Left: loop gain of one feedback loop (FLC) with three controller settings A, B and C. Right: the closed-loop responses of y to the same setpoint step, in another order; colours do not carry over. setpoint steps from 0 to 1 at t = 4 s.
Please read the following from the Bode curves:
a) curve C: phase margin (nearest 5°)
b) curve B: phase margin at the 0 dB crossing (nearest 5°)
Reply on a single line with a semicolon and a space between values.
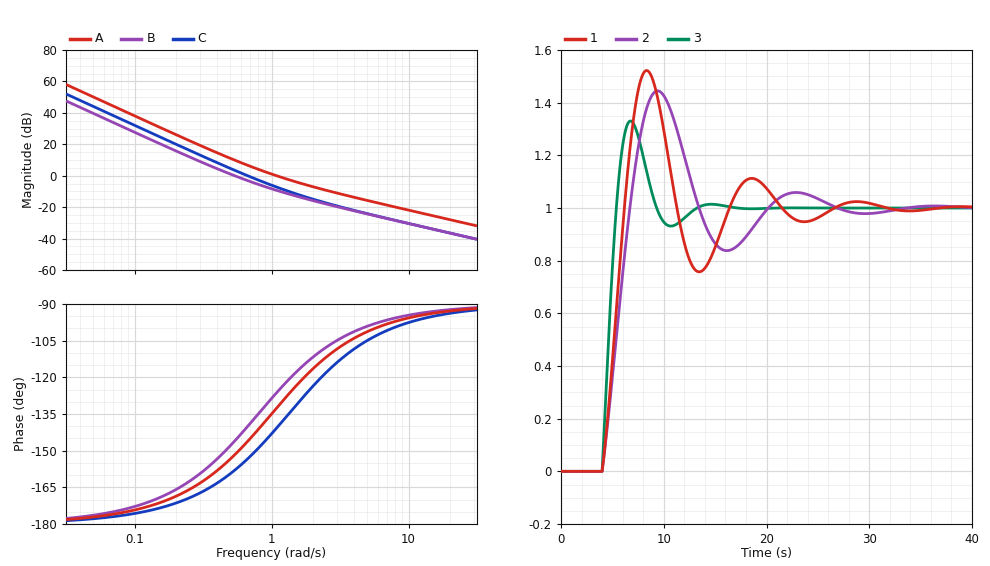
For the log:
25°; 35°
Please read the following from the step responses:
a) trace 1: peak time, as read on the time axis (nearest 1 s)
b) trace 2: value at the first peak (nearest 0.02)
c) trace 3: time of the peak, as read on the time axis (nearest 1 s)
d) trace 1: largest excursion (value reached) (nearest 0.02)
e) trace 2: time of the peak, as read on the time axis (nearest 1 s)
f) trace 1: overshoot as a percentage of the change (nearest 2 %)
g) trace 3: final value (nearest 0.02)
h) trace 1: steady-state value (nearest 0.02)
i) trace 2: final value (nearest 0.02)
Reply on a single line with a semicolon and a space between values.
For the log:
8 s; 1.44; 7 s; 1.52; 9 s; 52 %; 1.00; 1.00; 1.00
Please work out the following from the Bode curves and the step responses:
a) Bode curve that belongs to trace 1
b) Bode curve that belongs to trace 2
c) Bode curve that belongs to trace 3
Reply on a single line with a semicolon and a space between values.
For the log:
C; B; A
